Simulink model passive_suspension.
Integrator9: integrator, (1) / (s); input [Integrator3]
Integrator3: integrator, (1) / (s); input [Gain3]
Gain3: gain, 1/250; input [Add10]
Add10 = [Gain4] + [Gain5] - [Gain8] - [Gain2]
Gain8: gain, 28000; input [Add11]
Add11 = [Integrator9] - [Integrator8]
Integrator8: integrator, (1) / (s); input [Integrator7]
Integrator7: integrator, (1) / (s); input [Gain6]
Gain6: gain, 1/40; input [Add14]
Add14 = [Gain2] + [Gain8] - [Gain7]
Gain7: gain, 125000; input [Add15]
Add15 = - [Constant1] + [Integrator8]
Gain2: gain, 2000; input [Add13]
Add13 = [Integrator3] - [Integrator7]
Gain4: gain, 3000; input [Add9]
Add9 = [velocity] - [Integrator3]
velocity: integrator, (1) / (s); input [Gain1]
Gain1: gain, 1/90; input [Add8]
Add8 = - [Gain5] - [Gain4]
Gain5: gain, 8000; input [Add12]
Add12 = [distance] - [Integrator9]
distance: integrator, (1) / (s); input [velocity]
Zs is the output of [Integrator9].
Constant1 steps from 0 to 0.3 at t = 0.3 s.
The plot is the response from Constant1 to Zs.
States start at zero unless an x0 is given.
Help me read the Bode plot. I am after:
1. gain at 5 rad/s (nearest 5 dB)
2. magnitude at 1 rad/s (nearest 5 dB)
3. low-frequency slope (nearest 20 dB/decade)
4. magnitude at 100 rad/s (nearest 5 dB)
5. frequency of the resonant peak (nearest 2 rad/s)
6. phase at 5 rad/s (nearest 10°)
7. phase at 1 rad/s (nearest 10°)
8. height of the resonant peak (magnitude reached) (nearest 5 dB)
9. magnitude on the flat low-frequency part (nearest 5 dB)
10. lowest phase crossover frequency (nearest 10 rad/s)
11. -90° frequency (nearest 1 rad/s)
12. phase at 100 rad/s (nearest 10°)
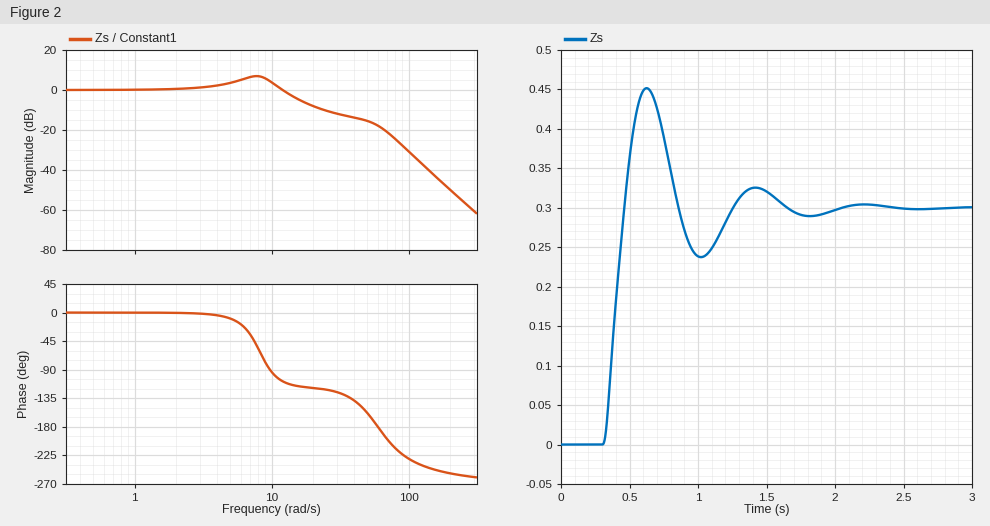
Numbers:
5 dB
0 dB
0 dB/decade
-30 dB
8 rad/s
-10°
0°
5 dB
0 dB
60 rad/s
10 rad/s
-230°
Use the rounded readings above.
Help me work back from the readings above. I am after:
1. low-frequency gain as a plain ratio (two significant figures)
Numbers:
1.0
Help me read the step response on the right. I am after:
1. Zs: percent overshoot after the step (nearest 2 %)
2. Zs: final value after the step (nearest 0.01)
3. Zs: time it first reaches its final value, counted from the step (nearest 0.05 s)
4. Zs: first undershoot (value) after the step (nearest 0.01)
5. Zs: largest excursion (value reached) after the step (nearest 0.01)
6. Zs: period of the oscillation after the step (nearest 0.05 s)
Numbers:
50 %
0.30
0.15 s
0.24
0.45
0.80 s
